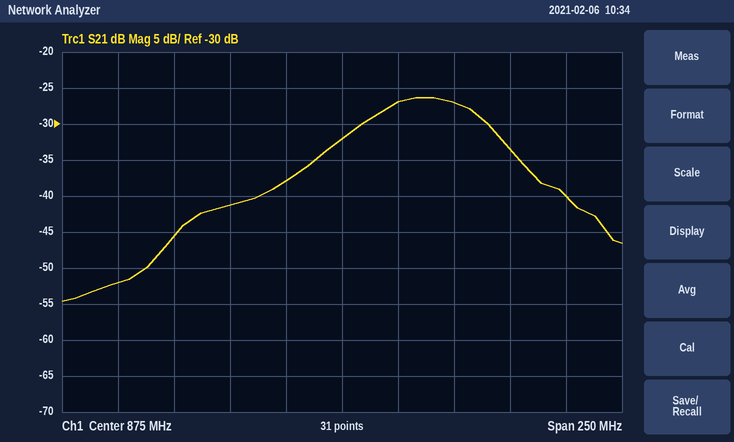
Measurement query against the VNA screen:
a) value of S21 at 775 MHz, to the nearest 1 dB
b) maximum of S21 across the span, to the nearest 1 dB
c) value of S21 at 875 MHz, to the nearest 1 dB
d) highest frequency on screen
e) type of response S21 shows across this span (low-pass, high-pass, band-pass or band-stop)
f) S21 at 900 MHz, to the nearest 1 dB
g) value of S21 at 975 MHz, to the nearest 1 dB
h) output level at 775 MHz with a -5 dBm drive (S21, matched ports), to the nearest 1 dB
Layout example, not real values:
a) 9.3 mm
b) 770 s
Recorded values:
a) -52 dB
b) -26 dB
c) -32 dB
d) 1 GHz
e) band-pass
f) -27 dB
g) -40 dB
h) -57 dBm
